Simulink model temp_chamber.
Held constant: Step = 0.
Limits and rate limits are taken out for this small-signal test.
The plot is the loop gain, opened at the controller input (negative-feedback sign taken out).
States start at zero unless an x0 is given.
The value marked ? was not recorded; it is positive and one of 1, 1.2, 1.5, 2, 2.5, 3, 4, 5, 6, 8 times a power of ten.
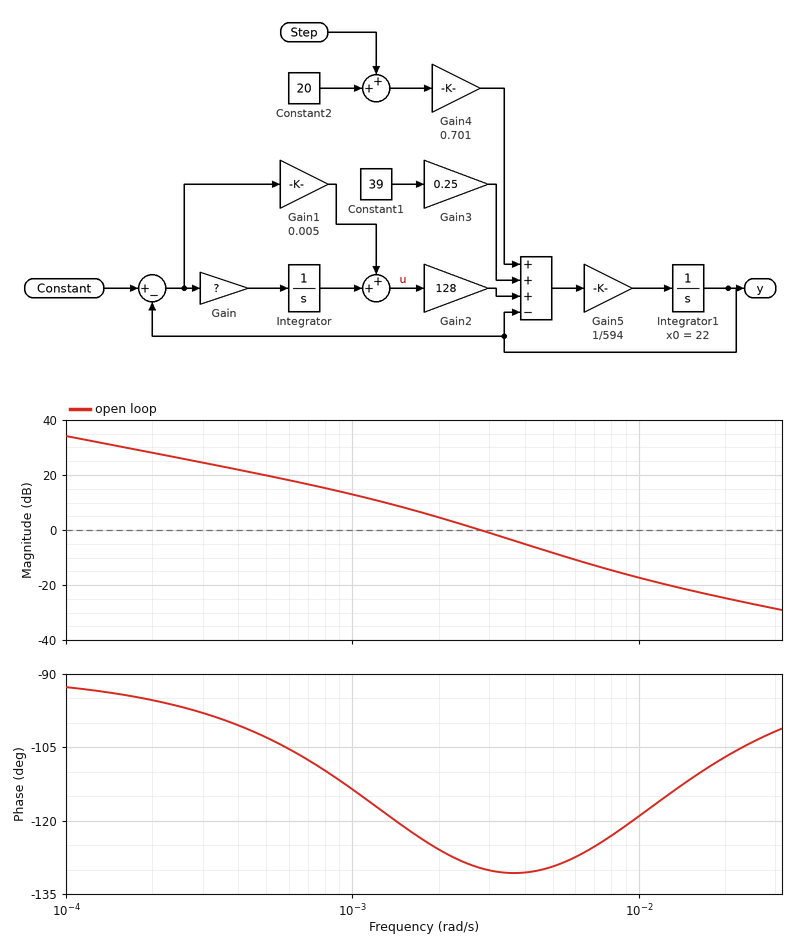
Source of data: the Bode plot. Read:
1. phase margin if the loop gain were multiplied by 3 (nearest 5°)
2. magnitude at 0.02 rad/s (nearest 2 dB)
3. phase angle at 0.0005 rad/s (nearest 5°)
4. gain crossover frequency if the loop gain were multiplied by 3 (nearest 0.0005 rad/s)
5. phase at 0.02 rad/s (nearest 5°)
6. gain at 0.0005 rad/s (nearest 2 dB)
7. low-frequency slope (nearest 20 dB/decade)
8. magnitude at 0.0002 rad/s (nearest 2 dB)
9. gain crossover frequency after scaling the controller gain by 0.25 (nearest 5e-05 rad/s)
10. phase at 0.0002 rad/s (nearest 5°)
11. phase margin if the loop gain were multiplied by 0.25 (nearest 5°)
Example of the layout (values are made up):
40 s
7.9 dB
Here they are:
50°
-24 dB
-105°
0.0055 rad/s
-105°
20 dB
-20 dB/decade
28 dB
0.00110 rad/s
-95°
65°
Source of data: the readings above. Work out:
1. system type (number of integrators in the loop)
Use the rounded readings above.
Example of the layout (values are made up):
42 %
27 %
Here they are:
1
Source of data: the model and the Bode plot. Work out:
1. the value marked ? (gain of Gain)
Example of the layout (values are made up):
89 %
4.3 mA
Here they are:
4e-05
